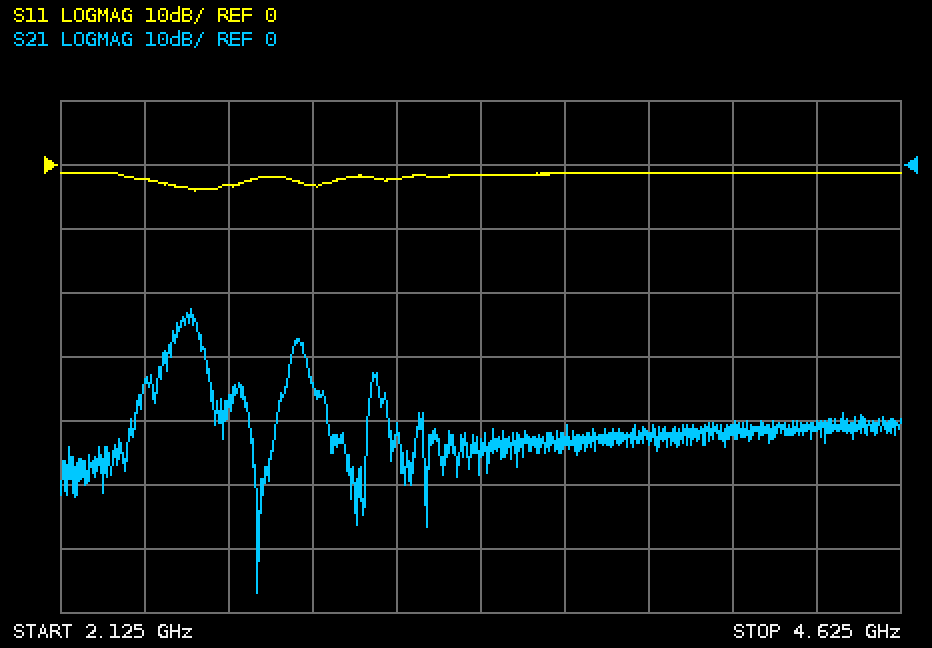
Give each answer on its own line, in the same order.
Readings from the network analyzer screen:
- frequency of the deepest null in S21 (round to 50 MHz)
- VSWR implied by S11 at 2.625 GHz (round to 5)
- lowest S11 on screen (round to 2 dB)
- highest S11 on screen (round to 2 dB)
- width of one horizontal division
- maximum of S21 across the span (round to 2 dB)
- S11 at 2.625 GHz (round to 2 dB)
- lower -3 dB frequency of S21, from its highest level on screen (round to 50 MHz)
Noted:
2.70 GHz
5
-4 dB
-2 dB
250 MHz
-22 dB
-4 dB
2.50 GHz
